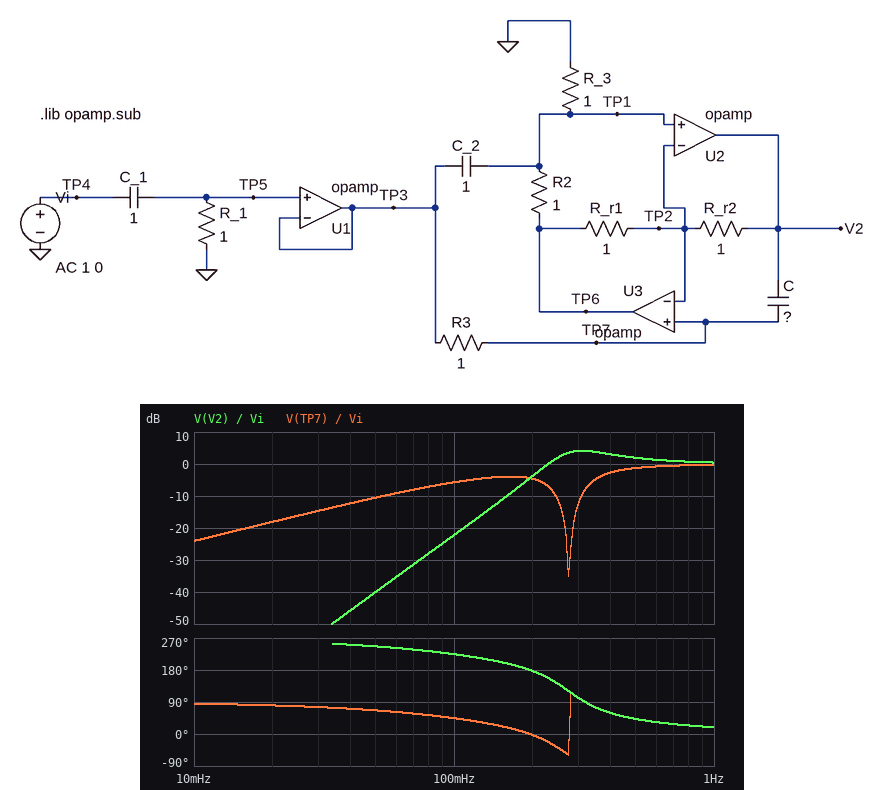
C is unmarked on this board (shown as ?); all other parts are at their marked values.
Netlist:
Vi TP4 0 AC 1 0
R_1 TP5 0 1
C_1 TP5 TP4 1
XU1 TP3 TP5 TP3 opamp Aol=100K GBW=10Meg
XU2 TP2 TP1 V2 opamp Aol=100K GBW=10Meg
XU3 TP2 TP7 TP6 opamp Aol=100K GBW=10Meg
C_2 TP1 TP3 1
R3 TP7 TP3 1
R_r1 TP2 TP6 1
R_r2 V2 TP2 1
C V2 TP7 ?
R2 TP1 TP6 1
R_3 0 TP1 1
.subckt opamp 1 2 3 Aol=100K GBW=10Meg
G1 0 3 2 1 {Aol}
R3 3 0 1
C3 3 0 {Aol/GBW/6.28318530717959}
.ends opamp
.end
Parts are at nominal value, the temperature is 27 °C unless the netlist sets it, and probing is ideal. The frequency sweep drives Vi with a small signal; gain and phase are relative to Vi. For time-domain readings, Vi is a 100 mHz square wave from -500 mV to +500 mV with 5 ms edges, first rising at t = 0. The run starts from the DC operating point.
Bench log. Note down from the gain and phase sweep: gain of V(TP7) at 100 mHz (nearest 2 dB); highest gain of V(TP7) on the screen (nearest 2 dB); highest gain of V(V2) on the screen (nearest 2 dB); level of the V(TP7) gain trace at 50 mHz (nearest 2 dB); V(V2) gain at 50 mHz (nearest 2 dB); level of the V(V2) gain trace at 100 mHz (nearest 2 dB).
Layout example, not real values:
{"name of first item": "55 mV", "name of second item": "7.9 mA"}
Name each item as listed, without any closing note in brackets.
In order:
{"gain of V(TP7) at 100 mHz": "-6 dB", "highest gain of V(TP7) on the screen": "0 dB", "highest gain of V(V2) on the screen": "4 dB", "level of the V(TP7) gain trace at 50 mHz": "-10 dB", "V(V2) gain at 50 mHz": "-40 dB", "level of the V(V2) gain trace at 100 mHz": "-22 dB"}
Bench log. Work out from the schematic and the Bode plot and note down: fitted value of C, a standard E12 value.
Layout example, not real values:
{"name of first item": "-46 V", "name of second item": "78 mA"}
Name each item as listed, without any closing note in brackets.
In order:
{"fitted value of C, a standard E12 value": "330 mF"}
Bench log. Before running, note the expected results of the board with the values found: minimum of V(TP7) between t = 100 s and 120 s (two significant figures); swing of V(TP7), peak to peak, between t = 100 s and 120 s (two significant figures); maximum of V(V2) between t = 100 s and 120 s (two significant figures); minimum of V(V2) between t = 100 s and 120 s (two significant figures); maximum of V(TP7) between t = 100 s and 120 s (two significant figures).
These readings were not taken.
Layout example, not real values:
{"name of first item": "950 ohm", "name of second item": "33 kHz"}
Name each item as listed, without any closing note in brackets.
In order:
{"minimum of V(TP7) between t = 100 s and 120 s": "-1.0 V", "swing of V(TP7), peak to peak, between t = 100 s and 120 s": "2.0 V", "maximum of V(V2) between t = 100 s and 120 s": "1.1 V", "minimum of V(V2) between t = 100 s and 120 s": "-1.1 V", "maximum of V(TP7) between t = 100 s and 120 s": "1.0 V"}
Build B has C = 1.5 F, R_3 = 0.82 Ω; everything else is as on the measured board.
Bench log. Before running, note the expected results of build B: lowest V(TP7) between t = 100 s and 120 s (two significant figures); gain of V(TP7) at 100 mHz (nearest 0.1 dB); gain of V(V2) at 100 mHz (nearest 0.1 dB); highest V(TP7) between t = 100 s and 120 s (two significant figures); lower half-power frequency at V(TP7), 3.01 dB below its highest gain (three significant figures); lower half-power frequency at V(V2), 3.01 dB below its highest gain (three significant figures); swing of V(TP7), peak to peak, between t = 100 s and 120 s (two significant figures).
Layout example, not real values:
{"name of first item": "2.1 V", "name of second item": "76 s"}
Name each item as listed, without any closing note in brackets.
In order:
{"lowest V(TP7) between t = 100 s and 120 s": "-850 mV", "gain of V(TP7) at 100 mHz": "-15.0 dB", "gain of V(V2) at 100 mHz": "-9.0 dB", "highest V(TP7) between t = 100 s and 120 s": "850 mV", "lower half-power frequency at V(TP7), 3.01 dB below its highest gain": "309 mHz", "lower half-power frequency at V(V2), 3.01 dB below its highest gain": "180 mHz", "swing of V(TP7), peak to peak, between t = 100 s and 120 s": "1.7 V"}
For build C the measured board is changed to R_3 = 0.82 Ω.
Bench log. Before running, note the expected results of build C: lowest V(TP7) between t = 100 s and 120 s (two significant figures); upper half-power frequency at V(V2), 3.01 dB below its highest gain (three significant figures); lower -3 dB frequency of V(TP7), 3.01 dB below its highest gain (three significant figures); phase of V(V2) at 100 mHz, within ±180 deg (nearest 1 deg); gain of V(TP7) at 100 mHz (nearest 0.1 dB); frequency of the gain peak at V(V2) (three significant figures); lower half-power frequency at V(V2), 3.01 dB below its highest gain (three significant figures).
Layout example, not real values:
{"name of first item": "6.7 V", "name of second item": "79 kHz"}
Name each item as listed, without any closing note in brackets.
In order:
{"lowest V(TP7) between t = 100 s and 120 s": "-1.0 V", "upper half-power frequency at V(V2), 3.01 dB below its highest gain": "730 mHz", "lower -3 dB frequency of V(TP7), 3.01 dB below its highest gain": "412 mHz", "phase of V(V2) at 100 mHz, within ±180 deg": "-138 deg", "gain of V(TP7) at 100 mHz": "-5.8 dB", "frequency of the gain peak at V(V2)": "314 mHz", "lower half-power frequency at V(V2), 3.01 dB below its highest gain": "229 mHz"}
